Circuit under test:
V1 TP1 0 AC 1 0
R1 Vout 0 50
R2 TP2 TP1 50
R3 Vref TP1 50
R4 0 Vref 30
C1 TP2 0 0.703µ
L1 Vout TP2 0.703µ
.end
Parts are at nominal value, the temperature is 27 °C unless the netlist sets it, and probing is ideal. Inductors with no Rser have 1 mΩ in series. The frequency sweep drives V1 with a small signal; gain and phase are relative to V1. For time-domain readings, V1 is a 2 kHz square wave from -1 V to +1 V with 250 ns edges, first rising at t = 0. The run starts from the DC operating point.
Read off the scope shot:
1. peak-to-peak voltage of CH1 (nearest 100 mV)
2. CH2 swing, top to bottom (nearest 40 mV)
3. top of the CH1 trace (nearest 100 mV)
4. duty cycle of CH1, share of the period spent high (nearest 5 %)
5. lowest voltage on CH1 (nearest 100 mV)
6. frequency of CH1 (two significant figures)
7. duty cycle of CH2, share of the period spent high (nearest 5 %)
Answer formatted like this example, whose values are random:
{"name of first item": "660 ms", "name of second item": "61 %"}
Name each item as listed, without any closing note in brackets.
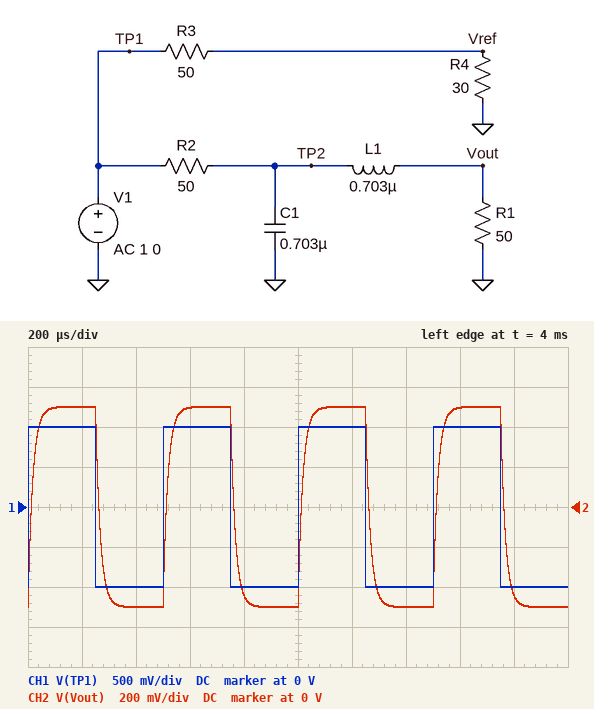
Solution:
{"peak-to-peak voltage of CH1": "2.0 V", "CH2 swing, top to bottom": "1.00 V", "top of the CH1 trace": "1.0 V", "duty cycle of CH1, share of the period spent high": "50 %", "lowest voltage on CH1": "-1.0 V", "frequency of CH1": "2.0 kHz", "duty cycle of CH2, share of the period spent high": "50 %"}
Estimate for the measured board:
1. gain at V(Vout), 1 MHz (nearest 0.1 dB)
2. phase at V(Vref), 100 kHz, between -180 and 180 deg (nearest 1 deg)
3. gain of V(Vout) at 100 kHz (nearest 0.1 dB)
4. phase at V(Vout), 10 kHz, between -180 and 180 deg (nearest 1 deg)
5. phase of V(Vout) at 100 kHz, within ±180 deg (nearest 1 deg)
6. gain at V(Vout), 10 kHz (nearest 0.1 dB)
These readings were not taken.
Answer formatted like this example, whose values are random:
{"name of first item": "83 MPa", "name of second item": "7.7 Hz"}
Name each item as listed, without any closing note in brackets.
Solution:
{"gain at V(Vout), 1 MHz": "-46.9 dB", "phase at V(Vref), 100 kHz, between -180 and 180 deg": "0 deg", "gain of V(Vout) at 100 kHz": "-26.9 dB", "phase at V(Vout), 10 kHz, between -180 and 180 deg": "-48 deg", "phase of V(Vout) at 100 kHz, within ±180 deg": "-85 deg", "gain at V(Vout), 10 kHz": "-9.5 dB"}
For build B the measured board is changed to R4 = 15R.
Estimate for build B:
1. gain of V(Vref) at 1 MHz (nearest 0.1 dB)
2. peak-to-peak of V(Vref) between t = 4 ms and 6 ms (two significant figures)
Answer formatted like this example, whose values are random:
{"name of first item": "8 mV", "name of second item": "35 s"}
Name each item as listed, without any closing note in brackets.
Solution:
{"gain of V(Vref) at 1 MHz": "-12.7 dB", "peak-to-peak of V(Vref) between t = 4 ms and 6 ms": "460 mV"}
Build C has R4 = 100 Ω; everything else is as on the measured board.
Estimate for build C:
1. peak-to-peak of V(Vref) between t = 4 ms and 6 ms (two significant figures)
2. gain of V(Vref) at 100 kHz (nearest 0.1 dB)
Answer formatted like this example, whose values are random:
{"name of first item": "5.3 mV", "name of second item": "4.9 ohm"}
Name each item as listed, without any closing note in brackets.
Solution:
{"peak-to-peak of V(Vref) between t = 4 ms and 6 ms": "1.3 V", "gain of V(Vref) at 100 kHz": "-3.5 dB"}
